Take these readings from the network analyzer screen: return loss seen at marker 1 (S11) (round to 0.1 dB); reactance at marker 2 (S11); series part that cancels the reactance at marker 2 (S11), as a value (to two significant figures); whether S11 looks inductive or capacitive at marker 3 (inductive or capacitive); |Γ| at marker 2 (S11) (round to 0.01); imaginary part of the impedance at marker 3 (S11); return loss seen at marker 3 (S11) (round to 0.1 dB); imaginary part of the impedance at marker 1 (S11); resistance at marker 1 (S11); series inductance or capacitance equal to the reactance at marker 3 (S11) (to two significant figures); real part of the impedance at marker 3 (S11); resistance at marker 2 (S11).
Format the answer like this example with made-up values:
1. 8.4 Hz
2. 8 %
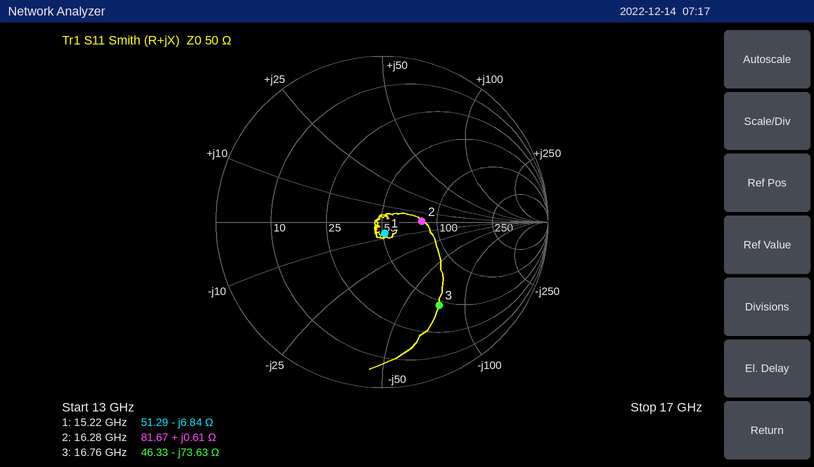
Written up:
1. 23.3 dB
2. +0.61 Ω
3. 16 pF
4. capacitive
5. 0.24
6. -73.63 Ω
7. 4.3 dB
8. -6.84 Ω
9. 51.29 Ω
10. 130 fF
11. 46.33 Ω
12. 81.67 Ω
